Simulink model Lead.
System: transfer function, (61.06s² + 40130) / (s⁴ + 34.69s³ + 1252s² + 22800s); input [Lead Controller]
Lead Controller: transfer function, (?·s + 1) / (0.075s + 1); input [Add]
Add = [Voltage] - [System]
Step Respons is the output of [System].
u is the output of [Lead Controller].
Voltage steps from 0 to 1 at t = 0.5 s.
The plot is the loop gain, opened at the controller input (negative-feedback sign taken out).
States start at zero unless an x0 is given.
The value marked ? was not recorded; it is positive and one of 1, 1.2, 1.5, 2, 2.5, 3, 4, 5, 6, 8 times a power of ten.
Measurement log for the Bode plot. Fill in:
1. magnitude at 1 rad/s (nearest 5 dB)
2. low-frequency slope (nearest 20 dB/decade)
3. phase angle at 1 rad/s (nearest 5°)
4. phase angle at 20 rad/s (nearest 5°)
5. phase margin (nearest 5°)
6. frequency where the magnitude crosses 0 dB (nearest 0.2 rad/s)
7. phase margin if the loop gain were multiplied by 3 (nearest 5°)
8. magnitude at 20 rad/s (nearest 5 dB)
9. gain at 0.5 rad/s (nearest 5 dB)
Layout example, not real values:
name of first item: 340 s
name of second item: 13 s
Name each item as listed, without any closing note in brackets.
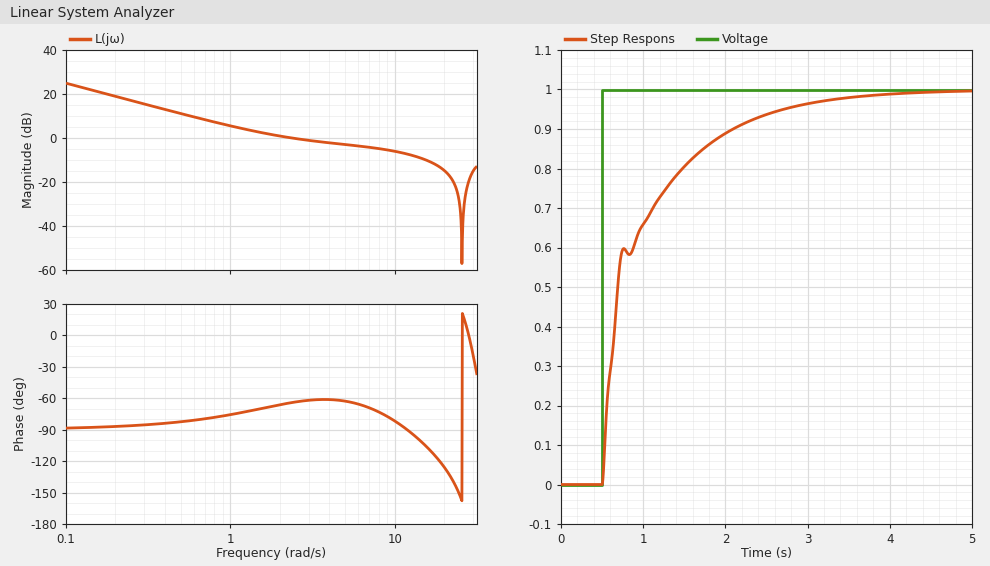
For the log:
magnitude at 1 rad/s: 5 dB
low-frequency slope: -20 dB/decade
phase angle at 1 rad/s: -75°
phase angle at 20 rad/s: -125°
phase margin: 115°
frequency where the magnitude crosses 0 dB: 2.4 rad/s
phase margin if the loop gain were multiplied by 3: 75°
magnitude at 20 rad/s: -15 dB
gain at 0.5 rad/s: 10 dB
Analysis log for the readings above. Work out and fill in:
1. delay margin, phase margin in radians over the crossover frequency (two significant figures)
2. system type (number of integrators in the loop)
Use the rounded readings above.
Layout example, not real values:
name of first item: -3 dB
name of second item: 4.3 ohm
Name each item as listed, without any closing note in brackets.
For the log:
delay margin, phase margin in radians over the crossover frequency: 0.84 s
system type: 1
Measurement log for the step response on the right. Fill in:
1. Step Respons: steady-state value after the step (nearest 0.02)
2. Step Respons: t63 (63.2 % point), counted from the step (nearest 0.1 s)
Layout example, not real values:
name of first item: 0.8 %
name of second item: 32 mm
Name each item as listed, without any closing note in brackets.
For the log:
Step Respons: steady-state value after the step: 1.00
Step Respons: t63 (63.2 % point), counted from the step: 0.4 s
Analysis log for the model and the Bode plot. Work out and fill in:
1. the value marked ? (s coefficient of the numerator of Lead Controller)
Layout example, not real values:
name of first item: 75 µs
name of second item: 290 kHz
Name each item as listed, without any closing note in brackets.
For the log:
the value marked ?: 0.4
